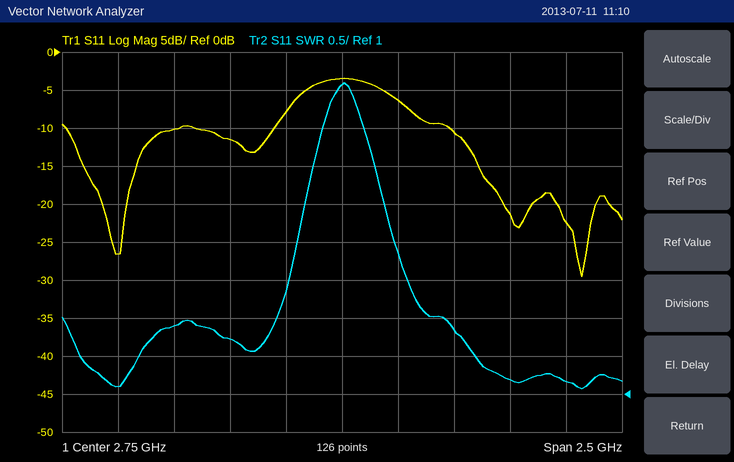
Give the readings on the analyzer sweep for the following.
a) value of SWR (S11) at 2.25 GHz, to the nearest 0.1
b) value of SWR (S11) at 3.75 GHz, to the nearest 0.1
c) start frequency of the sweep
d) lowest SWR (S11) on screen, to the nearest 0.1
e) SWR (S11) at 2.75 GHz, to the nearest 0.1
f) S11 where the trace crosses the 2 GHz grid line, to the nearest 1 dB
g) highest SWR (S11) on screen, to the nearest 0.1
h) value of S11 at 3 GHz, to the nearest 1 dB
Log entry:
1.7
1.2
1.5 GHz
1.1
5.1
-10 dB
5.1
-6 dB
